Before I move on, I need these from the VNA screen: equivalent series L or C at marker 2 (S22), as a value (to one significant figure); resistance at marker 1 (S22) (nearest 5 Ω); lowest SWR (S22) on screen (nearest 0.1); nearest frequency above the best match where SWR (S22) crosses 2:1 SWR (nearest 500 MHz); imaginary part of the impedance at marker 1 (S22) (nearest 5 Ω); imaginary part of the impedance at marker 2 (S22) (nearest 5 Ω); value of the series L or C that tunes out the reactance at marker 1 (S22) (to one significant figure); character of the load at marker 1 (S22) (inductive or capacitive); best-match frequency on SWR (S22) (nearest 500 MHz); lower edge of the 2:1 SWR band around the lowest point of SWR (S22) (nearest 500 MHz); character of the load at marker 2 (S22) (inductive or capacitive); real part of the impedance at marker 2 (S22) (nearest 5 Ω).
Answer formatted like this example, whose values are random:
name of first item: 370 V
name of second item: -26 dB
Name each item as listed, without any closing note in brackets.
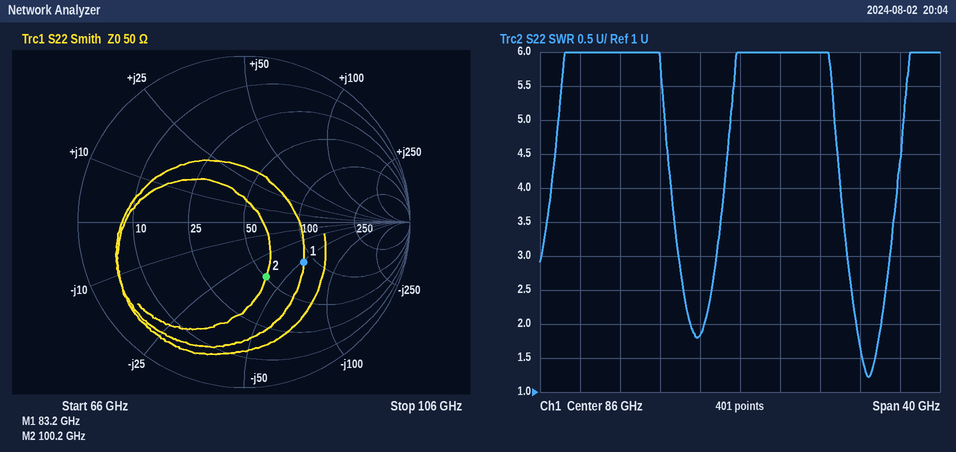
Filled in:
equivalent series L or C at marker 2 (S22), as a value: 40 fF
resistance at marker 1 (S22): 85 Ω
lowest SWR (S22) on screen: 1.2
nearest frequency above the best match where SWR (S22) crosses 2:1 SWR: 100.0 GHz
imaginary part of the impedance at marker 1 (S22): -50 Ω
imaginary part of the impedance at marker 2 (S22): -40 Ω
value of the series L or C that tunes out the reactance at marker 1 (S22): 100 pH
character of the load at marker 1 (S22): capacitive
best-match frequency on SWR (S22): 99.0 GHz
lower edge of the 2:1 SWR band around the lowest point of SWR (S22): 97.5 GHz
character of the load at marker 2 (S22): capacitive
real part of the impedance at marker 2 (S22): 50 Ω
